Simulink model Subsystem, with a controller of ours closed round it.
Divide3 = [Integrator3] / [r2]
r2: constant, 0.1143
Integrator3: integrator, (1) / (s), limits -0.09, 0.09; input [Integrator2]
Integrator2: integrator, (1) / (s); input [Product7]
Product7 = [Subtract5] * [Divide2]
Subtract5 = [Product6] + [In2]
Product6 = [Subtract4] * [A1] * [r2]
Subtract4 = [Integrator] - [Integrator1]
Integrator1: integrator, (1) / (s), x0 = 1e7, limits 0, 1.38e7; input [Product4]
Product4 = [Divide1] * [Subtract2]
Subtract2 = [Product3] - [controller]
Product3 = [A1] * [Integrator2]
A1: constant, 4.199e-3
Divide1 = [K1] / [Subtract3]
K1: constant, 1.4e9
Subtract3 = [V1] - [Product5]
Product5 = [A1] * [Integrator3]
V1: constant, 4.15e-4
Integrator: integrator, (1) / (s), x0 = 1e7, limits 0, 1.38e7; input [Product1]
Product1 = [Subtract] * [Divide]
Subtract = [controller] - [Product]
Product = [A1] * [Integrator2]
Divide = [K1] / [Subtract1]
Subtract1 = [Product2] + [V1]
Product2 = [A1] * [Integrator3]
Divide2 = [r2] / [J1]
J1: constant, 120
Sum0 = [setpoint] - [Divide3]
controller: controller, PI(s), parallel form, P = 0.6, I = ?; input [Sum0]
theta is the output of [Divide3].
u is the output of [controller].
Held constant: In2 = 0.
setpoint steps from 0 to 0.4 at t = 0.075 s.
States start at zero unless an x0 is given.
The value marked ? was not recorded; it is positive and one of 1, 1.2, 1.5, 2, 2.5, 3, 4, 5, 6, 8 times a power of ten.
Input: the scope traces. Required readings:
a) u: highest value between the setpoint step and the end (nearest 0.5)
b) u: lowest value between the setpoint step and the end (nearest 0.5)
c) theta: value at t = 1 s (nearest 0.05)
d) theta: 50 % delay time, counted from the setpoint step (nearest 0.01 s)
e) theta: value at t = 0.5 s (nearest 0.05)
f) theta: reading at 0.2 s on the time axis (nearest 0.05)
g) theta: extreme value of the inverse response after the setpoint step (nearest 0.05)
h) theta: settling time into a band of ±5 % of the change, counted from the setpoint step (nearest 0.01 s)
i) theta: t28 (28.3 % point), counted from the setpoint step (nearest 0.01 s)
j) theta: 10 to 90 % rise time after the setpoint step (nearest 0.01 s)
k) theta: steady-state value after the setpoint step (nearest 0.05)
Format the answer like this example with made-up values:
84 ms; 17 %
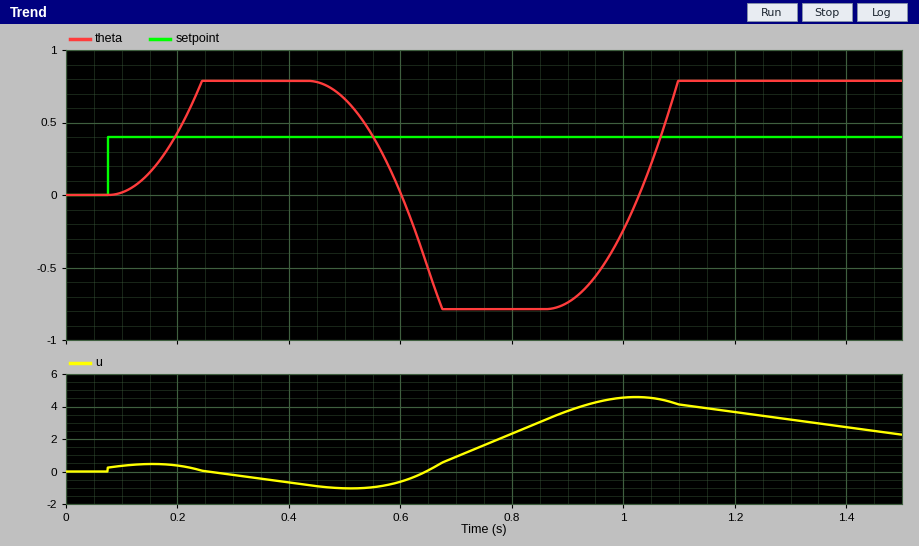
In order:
4.5; -1.0; -0.25; 0.12 s; 0.65; 0.45; -0.80; 1.02 s; 0.09 s; 0.11 s; 0.80
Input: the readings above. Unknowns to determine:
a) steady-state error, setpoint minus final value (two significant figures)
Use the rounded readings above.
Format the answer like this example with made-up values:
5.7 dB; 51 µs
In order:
-0.40
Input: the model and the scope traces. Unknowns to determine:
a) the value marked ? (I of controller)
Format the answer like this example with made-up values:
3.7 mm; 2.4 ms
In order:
12
